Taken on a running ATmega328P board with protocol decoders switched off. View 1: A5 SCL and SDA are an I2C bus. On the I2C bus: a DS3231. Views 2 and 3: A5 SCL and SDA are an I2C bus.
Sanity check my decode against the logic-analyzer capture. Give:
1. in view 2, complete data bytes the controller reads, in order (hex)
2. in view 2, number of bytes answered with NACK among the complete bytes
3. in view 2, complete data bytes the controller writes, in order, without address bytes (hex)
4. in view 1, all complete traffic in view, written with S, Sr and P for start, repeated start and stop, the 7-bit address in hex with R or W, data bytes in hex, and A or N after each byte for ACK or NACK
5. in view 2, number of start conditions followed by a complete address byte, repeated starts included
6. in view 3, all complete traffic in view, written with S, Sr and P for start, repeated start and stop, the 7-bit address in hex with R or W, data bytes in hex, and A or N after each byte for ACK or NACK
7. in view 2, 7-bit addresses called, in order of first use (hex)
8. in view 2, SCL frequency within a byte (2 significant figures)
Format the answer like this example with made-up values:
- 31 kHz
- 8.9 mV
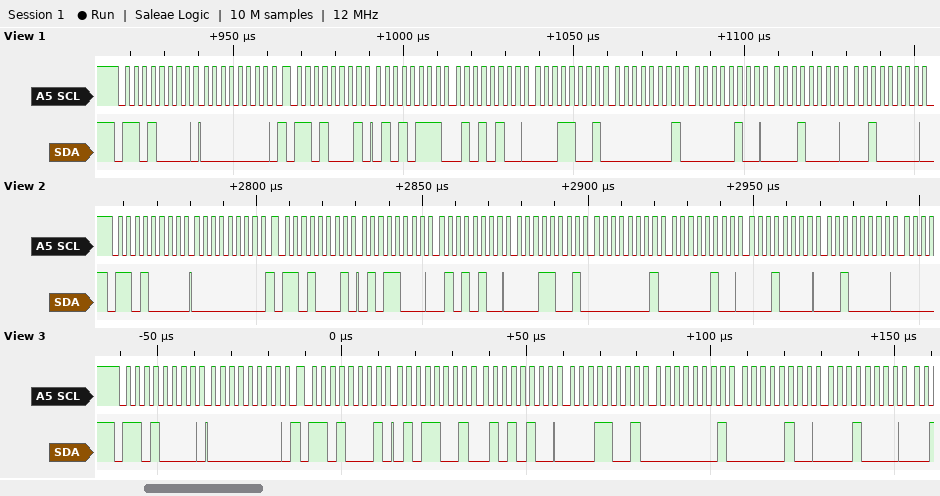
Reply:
- 58 54 19 01 04 10 20
- 0
- 00
- S 68W A 00 A Sr 68R A 57 A 54 A 19 A 01 A 04 A 10 A 20 A
- 2
- S 68W A 00 A Sr 68R A 59 A 54 A 19 A 01 A 04 A 10 A
- 0x68
- 400 kHz
